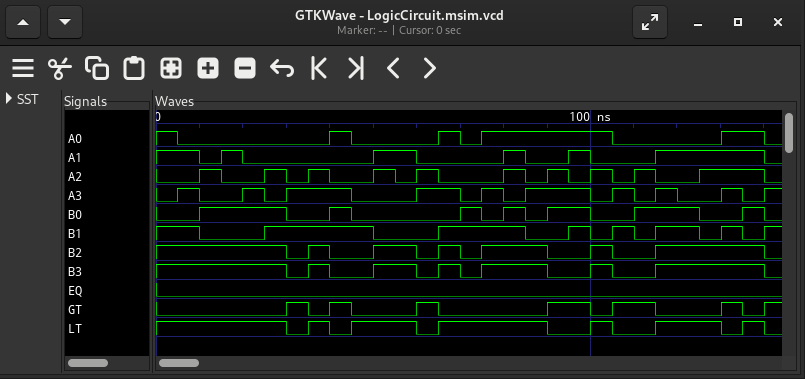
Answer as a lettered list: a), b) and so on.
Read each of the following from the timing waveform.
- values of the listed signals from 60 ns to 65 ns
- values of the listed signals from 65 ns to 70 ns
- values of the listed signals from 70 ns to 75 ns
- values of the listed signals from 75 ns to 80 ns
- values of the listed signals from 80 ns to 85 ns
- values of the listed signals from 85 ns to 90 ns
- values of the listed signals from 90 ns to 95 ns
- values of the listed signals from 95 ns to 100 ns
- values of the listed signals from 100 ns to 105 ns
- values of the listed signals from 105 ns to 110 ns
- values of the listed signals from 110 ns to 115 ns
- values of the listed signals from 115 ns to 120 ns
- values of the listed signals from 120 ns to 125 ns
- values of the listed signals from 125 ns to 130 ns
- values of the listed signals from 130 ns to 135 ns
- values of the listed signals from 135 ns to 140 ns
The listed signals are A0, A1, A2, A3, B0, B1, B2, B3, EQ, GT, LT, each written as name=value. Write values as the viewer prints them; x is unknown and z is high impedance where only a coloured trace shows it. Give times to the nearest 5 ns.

a) A0=0, A1=0, A2=1, A3=1, B0=0, B1=0, B2=0, B3=0, EQ=0, GT=1, LT=0
b) A0=1, A1=0, A2=0, A3=1, B0=0, B1=1, B2=1, B3=1, EQ=0, GT=0, LT=1
c) A0=0, A1=0, A2=0, A3=0, B0=1, B1=1, B2=0, B3=0, EQ=0, GT=0, LT=1
d) A0=1, A1=0, A2=0, A3=1, B0=0, B1=1, B2=1, B3=1, EQ=0, GT=0, LT=1
e) A0=1, A1=1, A2=1, A3=0, B0=1, B1=1, B2=1, B3=1, EQ=0, GT=0, LT=1
f) A0=1, A1=0, A2=0, A3=1, B0=0, B1=0, B2=1, B3=1, EQ=0, GT=0, LT=1
g) A0=1, A1=0, A2=1, A3=1, B0=1, B1=0, B2=0, B3=0, EQ=0, GT=1, LT=0
h) A0=1, A1=1, A2=0, A3=1, B0=1, B1=1, B2=0, B3=0, EQ=0, GT=1, LT=0
i) A0=1, A1=0, A2=1, A3=0, B0=0, B1=0, B2=1, B3=1, EQ=0, GT=0, LT=1
j) A0=0, A1=0, A2=0, A3=1, B0=0, B1=1, B2=0, B3=0, EQ=0, GT=1, LT=0
k) A0=0, A1=0, A2=1, A3=0, B0=1, B1=0, B2=0, B3=0, EQ=0, GT=1, LT=0
l) A0=0, A1=1, A2=0, A3=1, B0=1, B1=1, B2=1, B3=1, EQ=0, GT=0, LT=1
m) A0=0, A1=1, A2=0, A3=0, B0=1, B1=1, B2=1, B3=1, EQ=0, GT=0, LT=1
n) A0=0, A1=1, A2=1, A3=0, B0=0, B1=0, B2=1, B3=1, EQ=0, GT=0, LT=1
o) A0=1, A1=1, A2=1, A3=1, B0=0, B1=1, B2=1, B3=1, EQ=0, GT=1, LT=0
p) A0=1, A1=1, A2=1, A3=0, B0=1, B1=0, B2=1, B3=1, EQ=0, GT=0, LT=1
